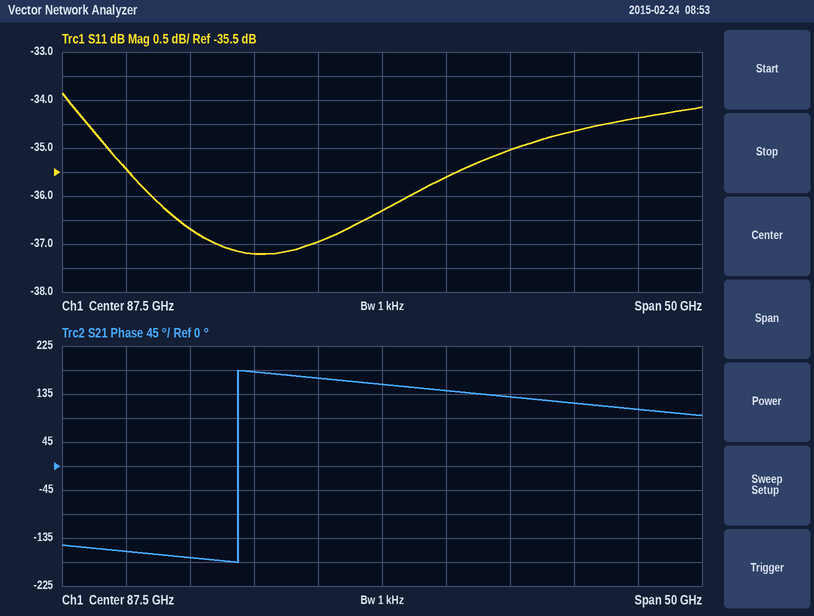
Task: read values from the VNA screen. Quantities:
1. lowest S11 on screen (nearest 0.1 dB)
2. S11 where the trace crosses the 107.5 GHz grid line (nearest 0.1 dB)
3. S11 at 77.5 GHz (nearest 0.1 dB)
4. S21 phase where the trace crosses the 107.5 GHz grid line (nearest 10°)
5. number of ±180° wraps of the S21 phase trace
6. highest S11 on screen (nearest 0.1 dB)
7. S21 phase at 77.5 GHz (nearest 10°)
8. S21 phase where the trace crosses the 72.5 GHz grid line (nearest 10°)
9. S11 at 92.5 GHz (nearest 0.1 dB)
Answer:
-37.2 dB
-34.4 dB
-37.2 dB
110°
1
-33.9 dB
180°
-170°
-35.6 dB
